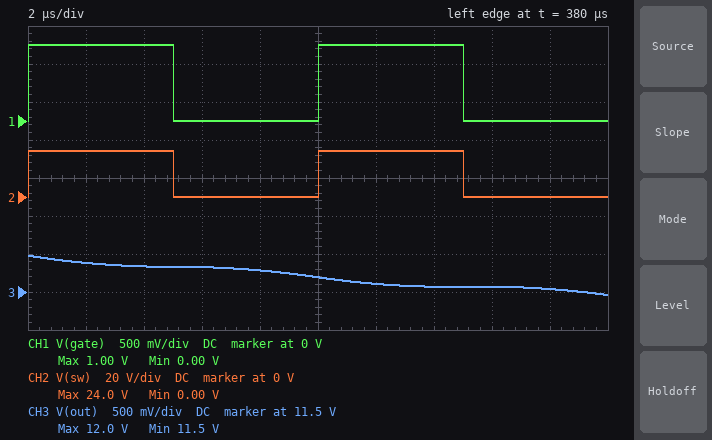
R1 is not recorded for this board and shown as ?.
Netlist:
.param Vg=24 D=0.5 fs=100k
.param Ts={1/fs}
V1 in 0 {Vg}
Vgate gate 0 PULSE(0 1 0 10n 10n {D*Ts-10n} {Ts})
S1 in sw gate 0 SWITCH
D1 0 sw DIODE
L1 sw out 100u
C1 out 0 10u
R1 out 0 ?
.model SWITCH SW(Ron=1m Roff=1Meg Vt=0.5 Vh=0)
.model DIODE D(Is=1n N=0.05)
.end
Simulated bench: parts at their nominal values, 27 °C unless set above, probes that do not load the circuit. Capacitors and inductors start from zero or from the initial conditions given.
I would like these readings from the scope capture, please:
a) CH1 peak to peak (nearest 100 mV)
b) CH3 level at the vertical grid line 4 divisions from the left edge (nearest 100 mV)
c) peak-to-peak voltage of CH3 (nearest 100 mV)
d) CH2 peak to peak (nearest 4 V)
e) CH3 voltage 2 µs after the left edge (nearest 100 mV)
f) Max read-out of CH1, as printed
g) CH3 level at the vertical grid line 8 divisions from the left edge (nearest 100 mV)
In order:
1.0 V
11.8 V
500 mV
24 V
11.9 V
1.00 V
11.6 V
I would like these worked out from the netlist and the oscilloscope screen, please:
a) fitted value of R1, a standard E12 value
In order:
12 Ω
